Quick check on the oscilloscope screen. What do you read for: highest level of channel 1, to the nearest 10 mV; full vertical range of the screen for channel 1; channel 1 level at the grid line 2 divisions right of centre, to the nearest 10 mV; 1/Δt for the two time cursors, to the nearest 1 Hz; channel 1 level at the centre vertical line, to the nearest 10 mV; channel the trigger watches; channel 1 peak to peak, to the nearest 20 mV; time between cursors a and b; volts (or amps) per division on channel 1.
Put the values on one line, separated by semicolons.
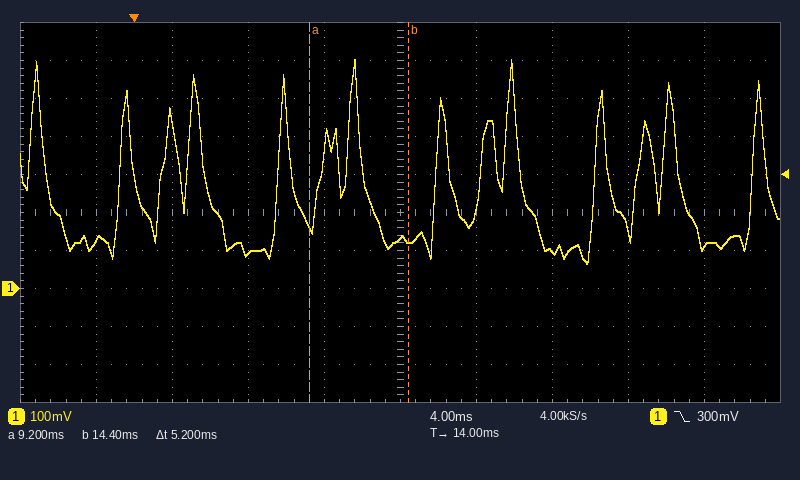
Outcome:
600 mV; 1 V; 100 mV; 192 Hz; 130 mV; channel 1; 540 mV; 5.2 ms; 100 mV
